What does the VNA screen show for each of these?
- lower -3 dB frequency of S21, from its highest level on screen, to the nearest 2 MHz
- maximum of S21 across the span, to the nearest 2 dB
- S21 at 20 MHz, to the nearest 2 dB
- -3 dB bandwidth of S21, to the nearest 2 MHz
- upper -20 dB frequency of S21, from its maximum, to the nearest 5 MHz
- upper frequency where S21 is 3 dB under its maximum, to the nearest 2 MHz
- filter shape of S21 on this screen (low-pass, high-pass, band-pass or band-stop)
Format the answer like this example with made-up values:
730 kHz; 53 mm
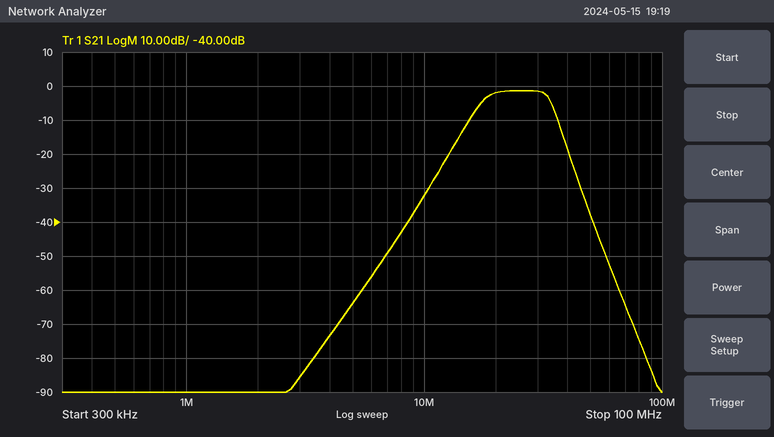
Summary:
18 MHz; -2 dB; -2 dB; 16 MHz; 40 MHz; 34 MHz; band-pass
